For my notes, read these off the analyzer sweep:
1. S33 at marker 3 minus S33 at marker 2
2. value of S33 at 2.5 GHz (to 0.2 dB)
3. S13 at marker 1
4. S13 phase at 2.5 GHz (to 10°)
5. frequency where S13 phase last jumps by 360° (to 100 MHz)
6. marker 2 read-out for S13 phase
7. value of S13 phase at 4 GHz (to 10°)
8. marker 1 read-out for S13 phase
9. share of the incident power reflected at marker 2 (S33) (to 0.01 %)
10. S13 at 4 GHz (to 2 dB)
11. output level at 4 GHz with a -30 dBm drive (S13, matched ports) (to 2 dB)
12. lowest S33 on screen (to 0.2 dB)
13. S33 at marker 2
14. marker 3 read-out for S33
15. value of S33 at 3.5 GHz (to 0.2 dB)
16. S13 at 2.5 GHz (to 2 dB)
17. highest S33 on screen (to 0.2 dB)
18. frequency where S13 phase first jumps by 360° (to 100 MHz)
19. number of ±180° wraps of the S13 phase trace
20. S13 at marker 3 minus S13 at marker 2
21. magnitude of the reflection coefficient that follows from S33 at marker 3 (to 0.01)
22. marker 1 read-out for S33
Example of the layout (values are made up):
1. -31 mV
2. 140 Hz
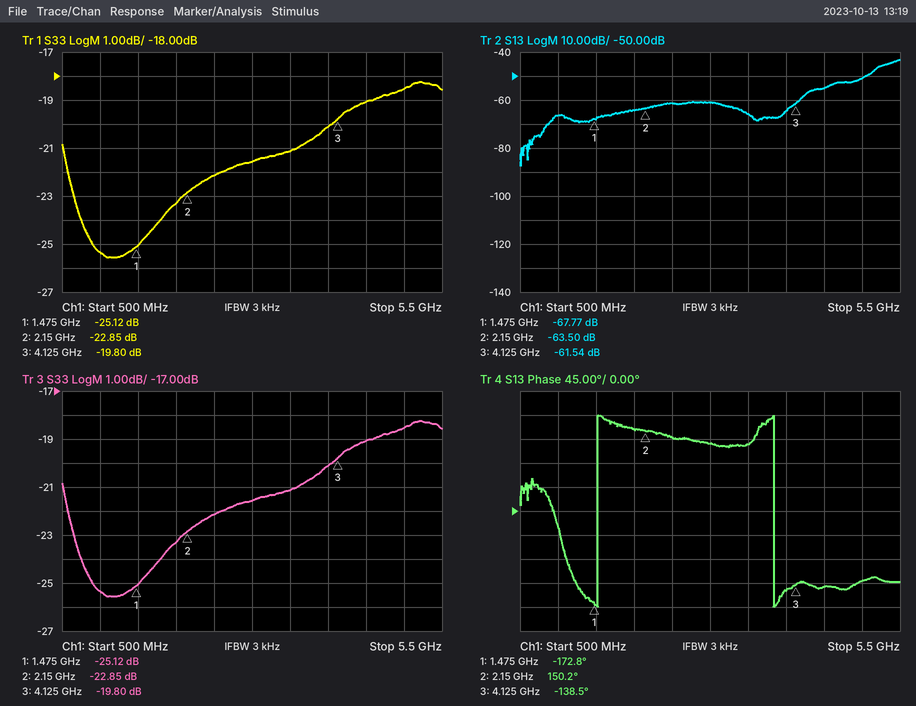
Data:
1. 3.05 dB
2. -22.2 dB
3. -67.77 dB
4. 140°
5. 3.8 GHz
6. 150.2°
7. -150°
8. -172.8°
9. 0.52 %
10. -64 dB
11. -94 dBm
12. -25.6 dB
13. -22.85 dB
14. -19.80 dB
15. -21.2 dB
16. -62 dB
17. -18.2 dB
18. 1.5 GHz
19. 2
20. 1.96 dB
21. 0.10
22. -25.12 dB
